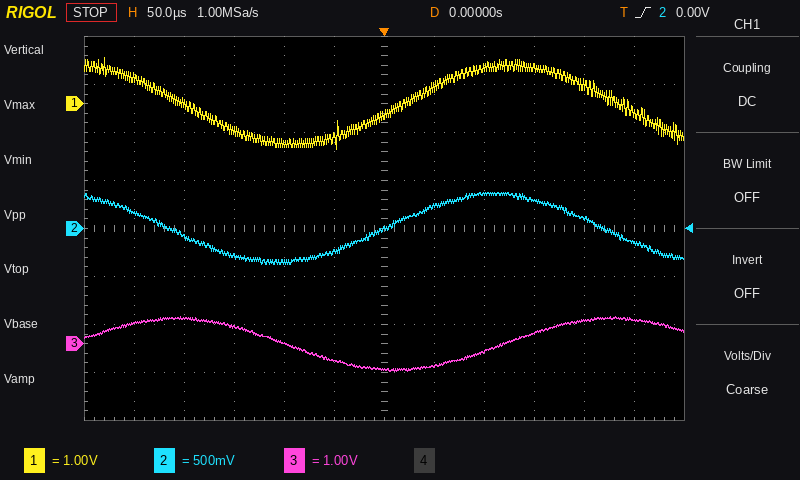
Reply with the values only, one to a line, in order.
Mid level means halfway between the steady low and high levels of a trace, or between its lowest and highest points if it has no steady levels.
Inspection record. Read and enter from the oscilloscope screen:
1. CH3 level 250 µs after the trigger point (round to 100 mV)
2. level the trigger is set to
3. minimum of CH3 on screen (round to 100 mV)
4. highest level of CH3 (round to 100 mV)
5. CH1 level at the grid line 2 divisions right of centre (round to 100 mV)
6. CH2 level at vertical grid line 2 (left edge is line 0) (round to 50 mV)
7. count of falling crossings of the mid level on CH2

500 mV
0.00 V
-600 mV
600 mV
700 mV
-100 mV
2
